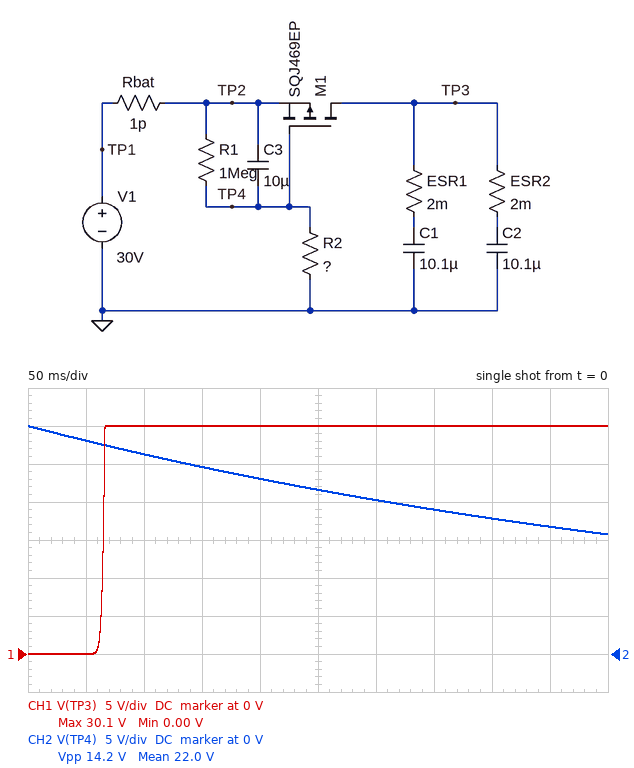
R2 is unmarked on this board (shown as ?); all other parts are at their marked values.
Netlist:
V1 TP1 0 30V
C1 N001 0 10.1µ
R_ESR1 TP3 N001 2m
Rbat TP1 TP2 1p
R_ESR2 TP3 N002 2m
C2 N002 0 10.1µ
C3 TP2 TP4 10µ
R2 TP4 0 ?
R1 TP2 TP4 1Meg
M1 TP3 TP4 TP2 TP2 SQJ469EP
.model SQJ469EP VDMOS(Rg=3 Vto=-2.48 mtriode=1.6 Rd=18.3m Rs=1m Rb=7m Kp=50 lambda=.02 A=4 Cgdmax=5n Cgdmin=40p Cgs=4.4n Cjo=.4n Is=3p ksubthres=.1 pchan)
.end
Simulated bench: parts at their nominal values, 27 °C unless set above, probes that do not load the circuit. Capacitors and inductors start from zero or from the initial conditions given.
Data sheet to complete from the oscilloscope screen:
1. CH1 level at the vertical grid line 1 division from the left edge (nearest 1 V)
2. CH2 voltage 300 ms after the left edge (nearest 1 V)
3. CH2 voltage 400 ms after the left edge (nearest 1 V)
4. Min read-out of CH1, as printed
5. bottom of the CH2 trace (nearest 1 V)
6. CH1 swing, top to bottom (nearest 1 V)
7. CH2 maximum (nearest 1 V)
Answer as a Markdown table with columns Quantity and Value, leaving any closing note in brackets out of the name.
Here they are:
| Quantity | Value |
|---|---|
| CH1 level at the vertical grid line 1 division from the left edge | 0 V |
| CH2 voltage 300 ms after the left edge | 20 V |
| CH2 voltage 400 ms after the left edge | 18 V |
| Min read-out of CH1, as printed | 0.00 V |
| bottom of the CH2 trace | 16 V |
| CH1 swing, top to bottom | 30 V |
| CH2 maximum | 30 V |
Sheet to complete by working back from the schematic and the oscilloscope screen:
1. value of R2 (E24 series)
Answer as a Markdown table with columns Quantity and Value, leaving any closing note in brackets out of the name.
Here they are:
| Quantity | Value |
|---|---|
| value of R2 | 75 kΩ |
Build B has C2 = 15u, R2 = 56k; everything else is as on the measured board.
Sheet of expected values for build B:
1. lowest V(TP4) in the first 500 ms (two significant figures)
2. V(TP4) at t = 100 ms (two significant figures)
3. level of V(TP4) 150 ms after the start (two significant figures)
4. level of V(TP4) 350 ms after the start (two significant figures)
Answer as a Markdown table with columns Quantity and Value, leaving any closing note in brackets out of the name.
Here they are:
| Quantity | Value |
|---|---|
| lowest V(TP4) in the first 500 ms | 13 V |
| V(TP4) at t = 100 ms | 25 V |
| level of V(TP4) 150 ms after the start | 23 V |
| level of V(TP4) 350 ms after the start | 16 V |
